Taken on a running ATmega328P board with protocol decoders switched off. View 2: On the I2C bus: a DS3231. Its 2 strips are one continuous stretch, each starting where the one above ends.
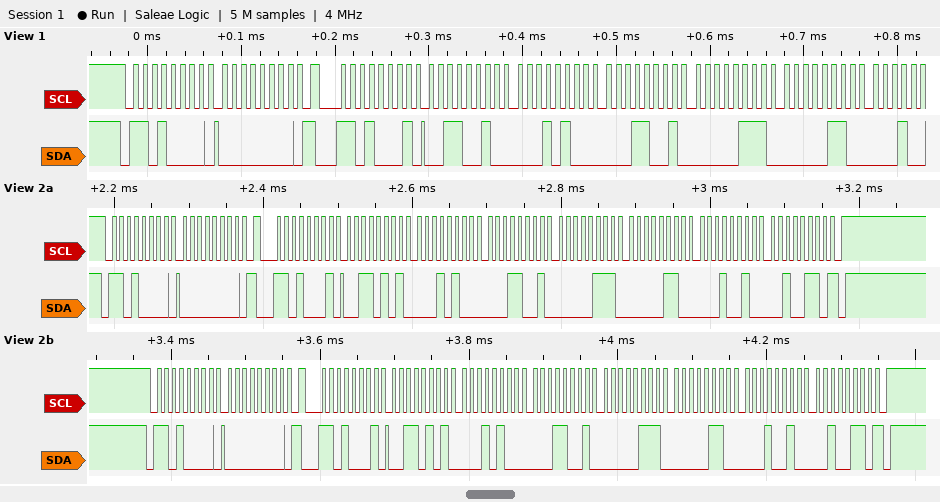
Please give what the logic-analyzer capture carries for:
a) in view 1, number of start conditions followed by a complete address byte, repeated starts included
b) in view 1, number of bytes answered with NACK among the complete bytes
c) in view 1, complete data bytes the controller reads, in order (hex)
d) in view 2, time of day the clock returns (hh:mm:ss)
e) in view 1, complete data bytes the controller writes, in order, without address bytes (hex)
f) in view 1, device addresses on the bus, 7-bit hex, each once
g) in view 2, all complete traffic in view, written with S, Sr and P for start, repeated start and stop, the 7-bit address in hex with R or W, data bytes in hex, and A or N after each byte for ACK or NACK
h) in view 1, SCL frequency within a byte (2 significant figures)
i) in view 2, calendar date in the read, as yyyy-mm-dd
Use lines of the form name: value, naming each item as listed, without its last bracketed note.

in view 1, number of start conditions followed by a complete address byte, repeated starts included: 2
in view 1, number of bytes answered with NACK among the complete bytes: 0
in view 1, complete data bytes the controller reads, in order: 32 14 19 07 06
in view 2, time of day the clock returns: 19:14:35
in view 1, complete data bytes the controller writes, in order, without address bytes: 00
in view 1, device addresses on the bus, 7-bit hex, each once: 0x68
in view 2, all complete traffic in view, written with S, Sr and P for start, repeated start and stop, the 7-bit address in hex with R or W, data bytes in hex, and A or N after each byte for ACK or NACK: S 68W A 00 A Sr 68R A 35 A 14 A 19 A 07 A 06 A 12 A 26 N P S 68W A 00 A Sr 68R A 35 A 14 A 19 A 07 A 06 A 12 A 26 N P
in view 1, SCL frequency within a byte: 100 kHz
in view 2, calendar date in the read, as yyyy-mm-dd: 2026-12-06
